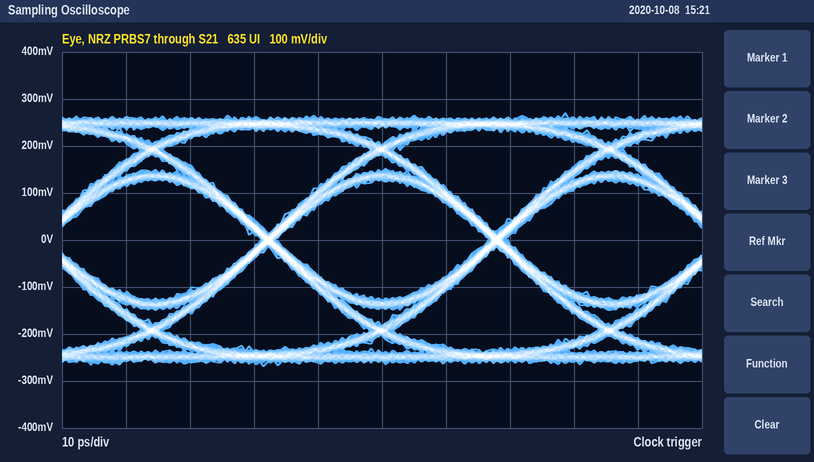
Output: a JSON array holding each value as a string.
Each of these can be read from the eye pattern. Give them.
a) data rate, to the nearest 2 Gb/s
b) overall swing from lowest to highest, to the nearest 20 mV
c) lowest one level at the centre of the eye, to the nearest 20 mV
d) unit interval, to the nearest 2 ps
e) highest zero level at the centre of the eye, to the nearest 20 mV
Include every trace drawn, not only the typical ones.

["28 Gb/s", "540 mV", "120 mV", "36 ps", "-120 mV"]
